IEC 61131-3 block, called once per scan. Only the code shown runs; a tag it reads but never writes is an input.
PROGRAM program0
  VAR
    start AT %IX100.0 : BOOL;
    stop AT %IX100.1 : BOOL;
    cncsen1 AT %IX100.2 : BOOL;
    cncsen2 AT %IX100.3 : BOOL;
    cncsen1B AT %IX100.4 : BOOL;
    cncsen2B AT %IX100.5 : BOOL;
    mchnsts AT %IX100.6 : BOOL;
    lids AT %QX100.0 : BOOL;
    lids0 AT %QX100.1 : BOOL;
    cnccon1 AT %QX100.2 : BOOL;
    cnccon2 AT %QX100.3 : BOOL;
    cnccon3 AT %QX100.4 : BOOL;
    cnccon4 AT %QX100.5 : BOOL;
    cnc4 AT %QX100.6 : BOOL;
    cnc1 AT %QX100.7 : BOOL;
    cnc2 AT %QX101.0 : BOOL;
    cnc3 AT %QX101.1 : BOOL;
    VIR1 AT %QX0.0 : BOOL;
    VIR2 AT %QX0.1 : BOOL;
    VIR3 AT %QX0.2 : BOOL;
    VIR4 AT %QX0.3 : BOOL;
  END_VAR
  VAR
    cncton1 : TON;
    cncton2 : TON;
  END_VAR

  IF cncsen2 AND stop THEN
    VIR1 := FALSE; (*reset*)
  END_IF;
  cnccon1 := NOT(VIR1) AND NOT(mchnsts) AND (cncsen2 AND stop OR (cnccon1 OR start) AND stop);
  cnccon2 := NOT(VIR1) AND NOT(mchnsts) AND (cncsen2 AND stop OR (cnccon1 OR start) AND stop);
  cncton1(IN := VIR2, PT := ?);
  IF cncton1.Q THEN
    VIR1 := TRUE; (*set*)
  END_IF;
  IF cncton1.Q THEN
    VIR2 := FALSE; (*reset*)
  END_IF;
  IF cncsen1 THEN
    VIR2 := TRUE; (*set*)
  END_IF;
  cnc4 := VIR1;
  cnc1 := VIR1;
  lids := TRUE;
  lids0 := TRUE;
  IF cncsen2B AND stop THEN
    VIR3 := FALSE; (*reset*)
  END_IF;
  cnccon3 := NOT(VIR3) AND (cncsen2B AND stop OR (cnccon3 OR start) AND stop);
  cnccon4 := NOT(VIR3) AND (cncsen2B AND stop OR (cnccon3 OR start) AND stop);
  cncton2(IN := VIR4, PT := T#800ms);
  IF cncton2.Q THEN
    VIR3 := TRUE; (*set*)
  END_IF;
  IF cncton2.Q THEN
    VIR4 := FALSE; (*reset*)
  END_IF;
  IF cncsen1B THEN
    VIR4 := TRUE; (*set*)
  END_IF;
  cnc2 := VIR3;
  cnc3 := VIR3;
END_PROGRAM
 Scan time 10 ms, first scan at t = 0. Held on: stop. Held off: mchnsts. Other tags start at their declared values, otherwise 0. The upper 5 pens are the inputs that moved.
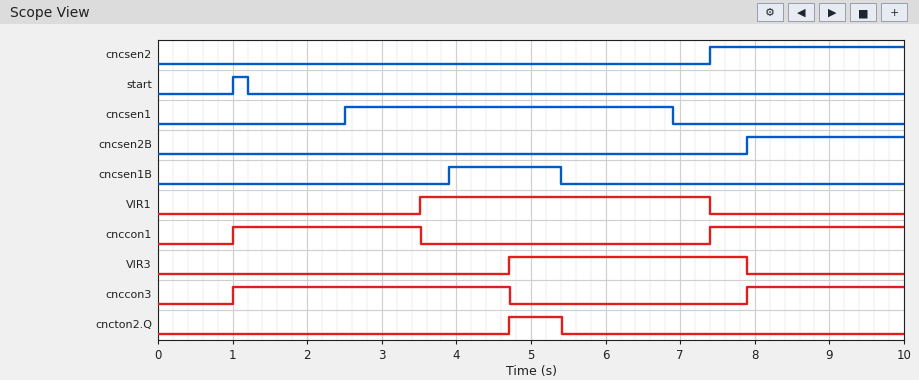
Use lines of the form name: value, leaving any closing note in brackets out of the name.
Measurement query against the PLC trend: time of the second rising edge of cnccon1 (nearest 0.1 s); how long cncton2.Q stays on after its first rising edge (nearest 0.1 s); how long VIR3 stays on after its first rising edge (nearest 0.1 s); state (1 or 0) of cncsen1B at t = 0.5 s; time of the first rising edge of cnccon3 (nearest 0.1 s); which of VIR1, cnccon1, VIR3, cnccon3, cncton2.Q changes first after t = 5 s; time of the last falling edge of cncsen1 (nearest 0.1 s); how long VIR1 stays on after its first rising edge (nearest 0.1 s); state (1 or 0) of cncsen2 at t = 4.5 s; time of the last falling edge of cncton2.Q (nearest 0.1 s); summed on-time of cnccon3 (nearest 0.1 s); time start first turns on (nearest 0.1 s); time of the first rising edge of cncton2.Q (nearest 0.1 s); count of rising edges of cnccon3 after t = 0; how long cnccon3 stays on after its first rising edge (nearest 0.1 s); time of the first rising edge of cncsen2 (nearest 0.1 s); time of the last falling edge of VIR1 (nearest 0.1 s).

time of the second rising edge of cnccon1: 7.4 s
how long cncton2.Q stays on after its first rising edge: 0.7 s
how long VIR3 stays on after its first rising edge: 3.2 s
state (1 or 0) of cncsen1B at t = 0.5 s: 0
time of the first rising edge of cnccon3: 1.0 s
which of VIR1, cnccon1, VIR3, cnccon3, cncton2.Q changes first after t = 5 s: cncton2.Q
time of the last falling edge of cncsen1: 6.9 s
how long VIR1 stays on after its first rising edge: 3.9 s
state (1 or 0) of cncsen2 at t = 4.5 s: 0
time of the last falling edge of cncton2.Q: 5.4 s
summed on-time of cnccon3: 5.8 s
time start first turns on: 1.0 s
time of the first rising edge of cncton2.Q: 4.7 s
count of rising edges of cnccon3 after t = 0: 2
how long cnccon3 stays on after its first rising edge: 3.7 s
time of the first rising edge of cncsen2: 7.4 s
time of the last falling edge of VIR1: 7.4 s
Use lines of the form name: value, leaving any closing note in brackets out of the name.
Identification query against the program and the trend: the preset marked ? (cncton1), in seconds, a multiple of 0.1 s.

the preset marked ? (cncton1), in seconds, a multiple of 0.1 s: 1.0 s
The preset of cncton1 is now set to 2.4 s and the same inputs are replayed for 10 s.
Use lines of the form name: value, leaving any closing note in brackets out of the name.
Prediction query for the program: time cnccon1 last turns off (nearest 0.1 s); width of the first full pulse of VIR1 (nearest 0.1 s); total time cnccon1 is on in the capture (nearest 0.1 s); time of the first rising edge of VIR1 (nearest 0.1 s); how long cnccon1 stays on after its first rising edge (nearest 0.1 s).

time cnccon1 last turns off: 4.9 s
width of the first full pulse of VIR1: 2.5 s
total time cnccon1 is on in the capture: 6.5 s
time of the first rising edge of VIR1: 4.9 s
how long cnccon1 stays on after its first rising edge: 3.9 s
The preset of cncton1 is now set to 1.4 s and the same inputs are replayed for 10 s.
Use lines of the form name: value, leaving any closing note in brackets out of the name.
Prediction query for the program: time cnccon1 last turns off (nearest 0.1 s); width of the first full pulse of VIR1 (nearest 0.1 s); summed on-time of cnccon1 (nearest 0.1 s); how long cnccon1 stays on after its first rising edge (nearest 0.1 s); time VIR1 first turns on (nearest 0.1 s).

time cnccon1 last turns off: 3.9 s
width of the first full pulse of VIR1: 3.5 s
summed on-time of cnccon1: 5.5 s
how long cnccon1 stays on after its first rising edge: 2.9 s
time VIR1 first turns on: 3.9 s
